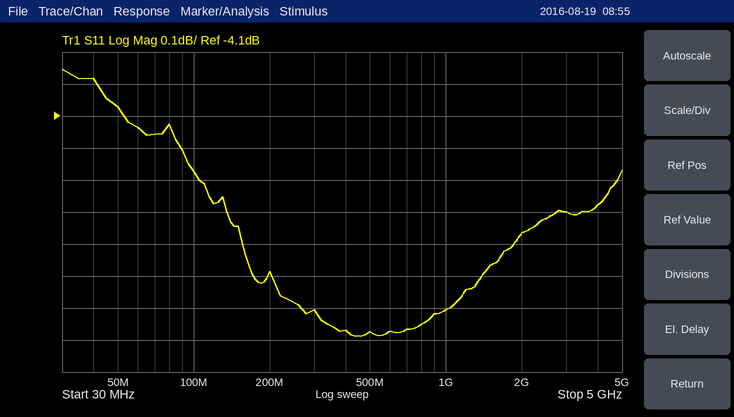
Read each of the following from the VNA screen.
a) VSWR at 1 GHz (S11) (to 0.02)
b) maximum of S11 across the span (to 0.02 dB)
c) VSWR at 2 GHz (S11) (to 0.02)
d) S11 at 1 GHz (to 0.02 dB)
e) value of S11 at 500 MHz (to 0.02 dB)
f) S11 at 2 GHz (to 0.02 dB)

3.78
-3.96 dB
3.98
-4.70 dB
-4.78 dB
-4.46 dB
